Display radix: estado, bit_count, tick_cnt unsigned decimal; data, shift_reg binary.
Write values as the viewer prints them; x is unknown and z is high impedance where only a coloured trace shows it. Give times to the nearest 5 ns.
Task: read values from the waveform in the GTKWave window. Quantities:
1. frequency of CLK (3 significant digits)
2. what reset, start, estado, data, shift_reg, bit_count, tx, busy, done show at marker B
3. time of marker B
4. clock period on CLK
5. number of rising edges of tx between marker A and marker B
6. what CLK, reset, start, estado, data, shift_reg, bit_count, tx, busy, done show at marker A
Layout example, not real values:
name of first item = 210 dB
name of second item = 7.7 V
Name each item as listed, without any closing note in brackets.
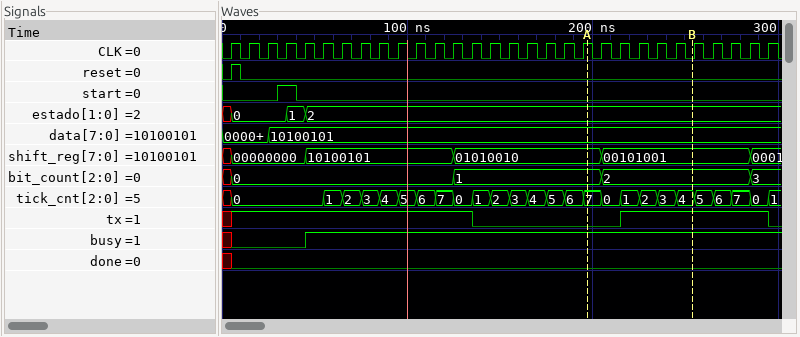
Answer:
frequency of CLK = 100 MHz
what reset, start, estado, data, shift_reg, bit_count, tx, busy, done show at marker B = reset=0, start=0, estado=2, data=10100101, shift_reg=00101001, bit_count=2, tx=1, busy=1, done=0
time of marker B = 255 ns
clock period on CLK = 10 ns
number of rising edges of tx between marker A and marker B = 1
what CLK, reset, start, estado, data, shift_reg, bit_count, tx, busy, done show at marker A = CLK=1, reset=0, start=0, estado=2, data=10100101, shift_reg=01010010, bit_count=1, tx=0, busy=1, done=0
